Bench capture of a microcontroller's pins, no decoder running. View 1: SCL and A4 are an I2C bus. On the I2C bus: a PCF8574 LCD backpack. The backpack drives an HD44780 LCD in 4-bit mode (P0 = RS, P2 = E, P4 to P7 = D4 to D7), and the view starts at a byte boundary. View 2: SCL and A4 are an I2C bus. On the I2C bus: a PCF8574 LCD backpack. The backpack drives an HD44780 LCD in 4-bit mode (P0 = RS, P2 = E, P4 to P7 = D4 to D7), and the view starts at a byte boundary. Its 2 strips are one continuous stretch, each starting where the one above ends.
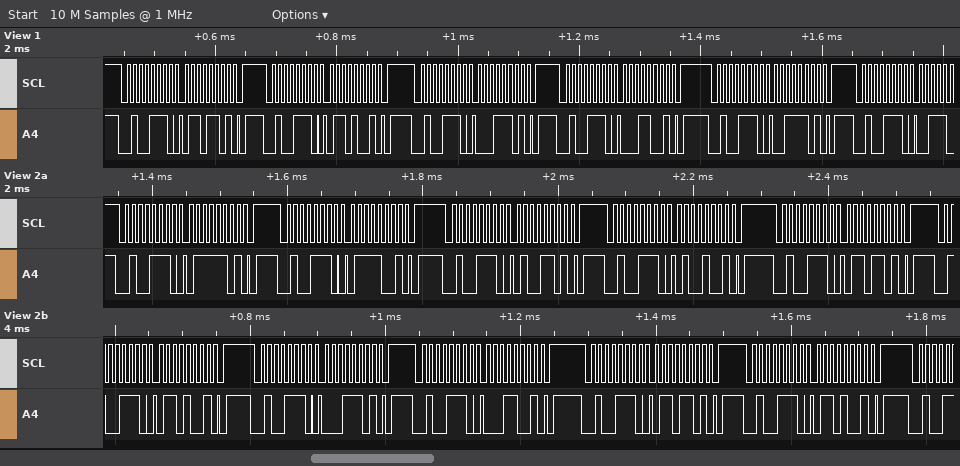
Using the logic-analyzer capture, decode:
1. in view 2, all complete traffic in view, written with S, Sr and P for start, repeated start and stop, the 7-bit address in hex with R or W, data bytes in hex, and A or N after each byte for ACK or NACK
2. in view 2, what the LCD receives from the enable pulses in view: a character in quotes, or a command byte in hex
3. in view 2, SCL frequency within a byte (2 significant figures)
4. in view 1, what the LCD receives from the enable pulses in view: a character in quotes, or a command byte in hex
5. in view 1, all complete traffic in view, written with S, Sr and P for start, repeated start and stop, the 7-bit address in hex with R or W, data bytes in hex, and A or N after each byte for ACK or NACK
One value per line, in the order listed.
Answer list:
S 27W A 7D A P S 27W A 79 A P S 27W A 4D A P S 27W A 49 A P S 27W A 6D A P S 27W A 69 A P S 27W A 1D A P S 27W A 19 A P S 27W A 6D A P S 27W A 69 A P
't' 'a'
100 kHz
'a'
S 27W A 6D A P S 27W A 69 A P S 27W A 1D A P S 27W A 19 A P S 27W A 3D A P S 27W A
